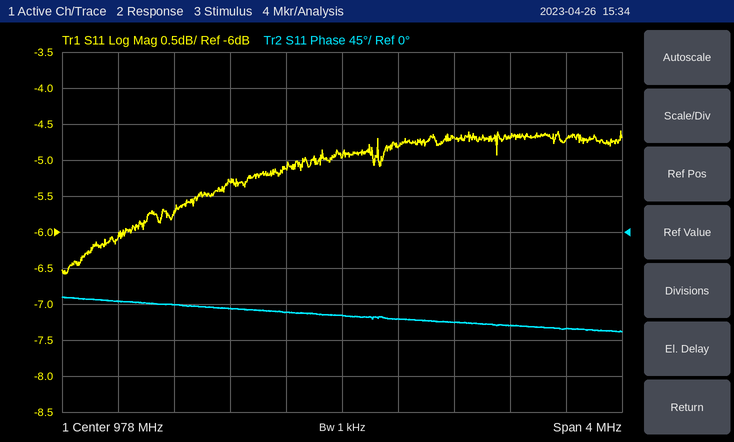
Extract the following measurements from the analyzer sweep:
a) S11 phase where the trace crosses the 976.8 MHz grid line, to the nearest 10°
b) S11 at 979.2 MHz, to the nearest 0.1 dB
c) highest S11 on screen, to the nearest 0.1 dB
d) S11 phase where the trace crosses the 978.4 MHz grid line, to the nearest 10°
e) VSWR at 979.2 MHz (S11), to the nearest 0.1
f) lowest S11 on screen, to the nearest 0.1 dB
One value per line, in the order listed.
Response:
-90°
-4.7 dB
-4.6 dB
-110°
3.8
-6.6 dB
